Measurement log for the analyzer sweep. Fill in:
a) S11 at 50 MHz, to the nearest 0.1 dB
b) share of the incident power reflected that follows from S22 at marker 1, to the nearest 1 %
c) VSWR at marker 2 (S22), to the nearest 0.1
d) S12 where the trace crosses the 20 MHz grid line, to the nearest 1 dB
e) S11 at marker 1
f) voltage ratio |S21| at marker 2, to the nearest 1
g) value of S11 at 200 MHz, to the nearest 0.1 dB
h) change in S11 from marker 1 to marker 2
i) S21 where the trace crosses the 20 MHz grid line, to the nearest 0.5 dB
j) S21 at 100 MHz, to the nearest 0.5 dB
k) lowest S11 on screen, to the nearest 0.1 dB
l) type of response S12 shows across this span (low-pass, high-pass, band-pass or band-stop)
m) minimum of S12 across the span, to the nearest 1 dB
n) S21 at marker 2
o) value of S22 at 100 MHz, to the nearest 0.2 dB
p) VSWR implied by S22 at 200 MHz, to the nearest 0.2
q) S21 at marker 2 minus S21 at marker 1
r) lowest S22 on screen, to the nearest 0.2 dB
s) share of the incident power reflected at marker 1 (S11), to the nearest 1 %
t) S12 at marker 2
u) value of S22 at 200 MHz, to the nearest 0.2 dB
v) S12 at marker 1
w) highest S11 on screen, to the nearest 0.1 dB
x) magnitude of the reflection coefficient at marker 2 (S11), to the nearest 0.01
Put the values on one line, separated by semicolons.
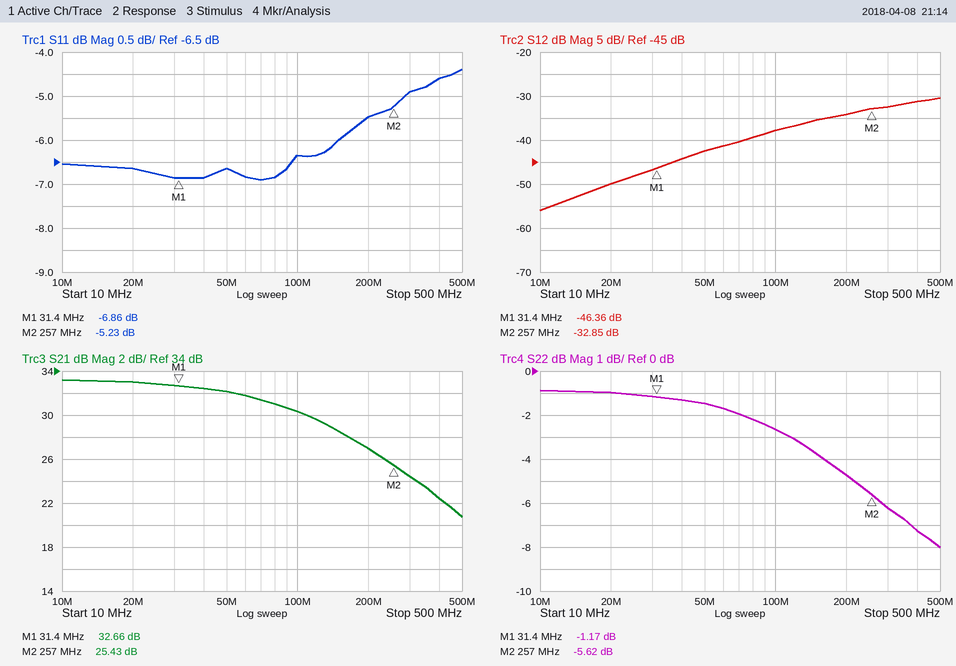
-6.6 dB; 76 %; 3.2; -50 dB; -6.86 dB; 19; -5.5 dB; 1.63 dB; 33.0 dB; 30.5 dB; -6.9 dB; high-pass; -56 dB; 25.43 dB; -2.6 dB; 3.8; -7.23 dB; -8.0 dB; 21 %; -32.85 dB; -4.8 dB; -46.36 dB; -4.4 dB; 0.55
